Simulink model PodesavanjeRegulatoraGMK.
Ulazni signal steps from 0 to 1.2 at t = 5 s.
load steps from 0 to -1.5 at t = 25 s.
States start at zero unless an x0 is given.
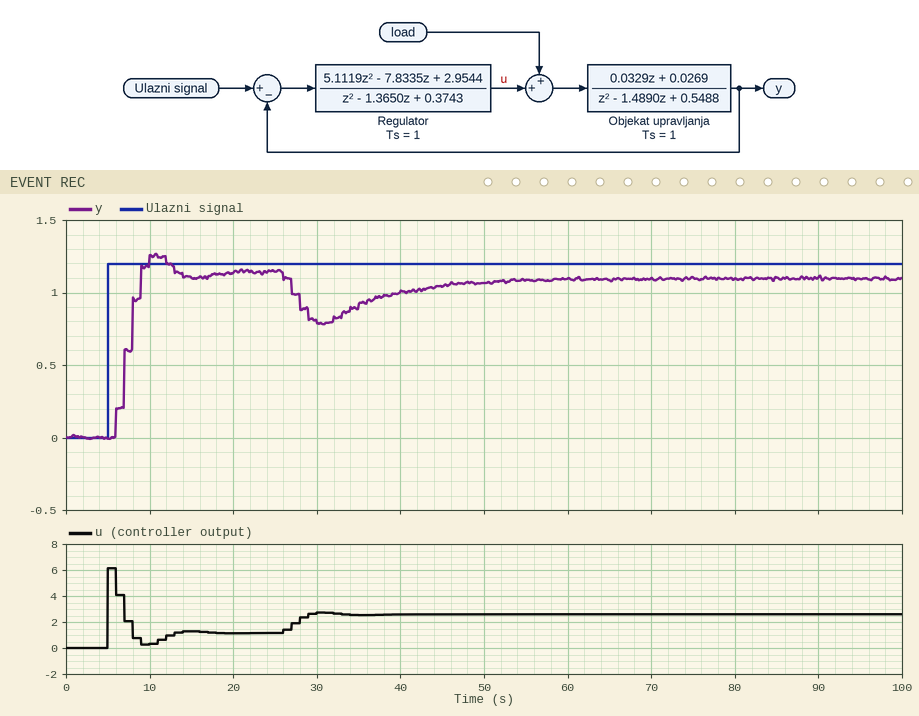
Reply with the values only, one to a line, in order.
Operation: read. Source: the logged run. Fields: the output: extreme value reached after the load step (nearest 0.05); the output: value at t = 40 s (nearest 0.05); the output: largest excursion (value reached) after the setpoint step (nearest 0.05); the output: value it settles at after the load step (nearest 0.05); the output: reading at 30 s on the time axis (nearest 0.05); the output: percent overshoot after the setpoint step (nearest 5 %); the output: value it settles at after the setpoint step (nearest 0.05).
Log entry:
0.80
1.00
1.25
1.10
0.80
10 %
1.15
